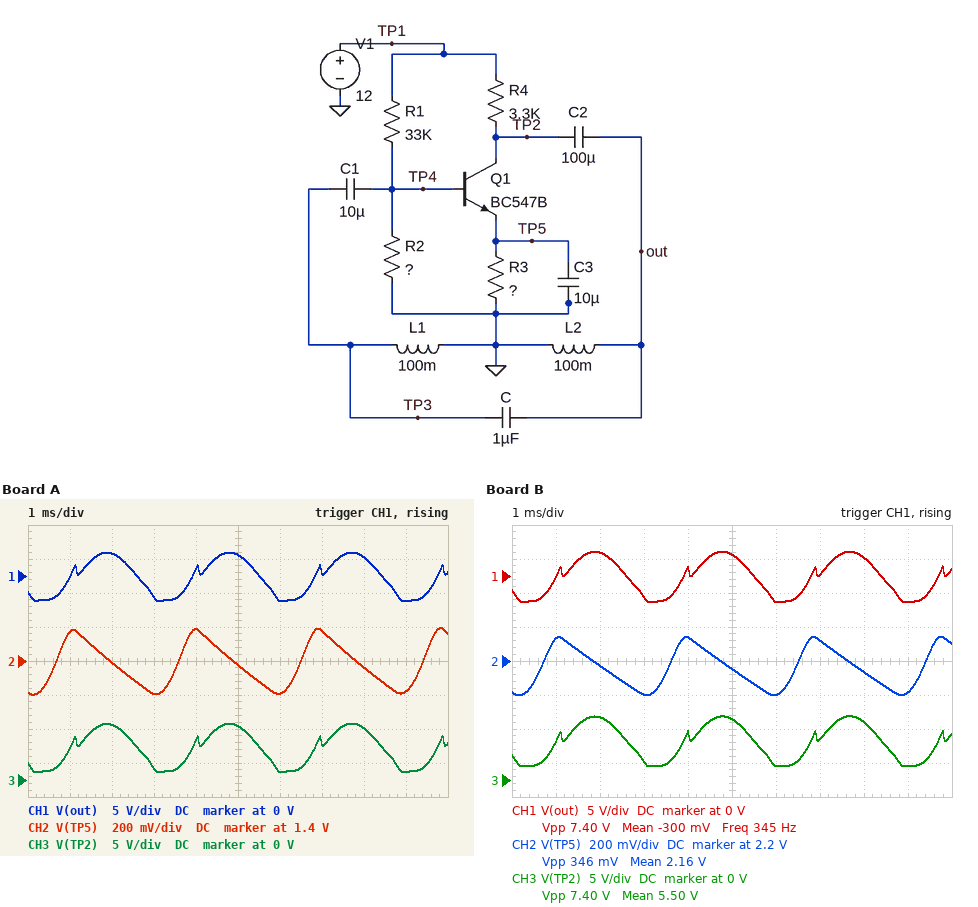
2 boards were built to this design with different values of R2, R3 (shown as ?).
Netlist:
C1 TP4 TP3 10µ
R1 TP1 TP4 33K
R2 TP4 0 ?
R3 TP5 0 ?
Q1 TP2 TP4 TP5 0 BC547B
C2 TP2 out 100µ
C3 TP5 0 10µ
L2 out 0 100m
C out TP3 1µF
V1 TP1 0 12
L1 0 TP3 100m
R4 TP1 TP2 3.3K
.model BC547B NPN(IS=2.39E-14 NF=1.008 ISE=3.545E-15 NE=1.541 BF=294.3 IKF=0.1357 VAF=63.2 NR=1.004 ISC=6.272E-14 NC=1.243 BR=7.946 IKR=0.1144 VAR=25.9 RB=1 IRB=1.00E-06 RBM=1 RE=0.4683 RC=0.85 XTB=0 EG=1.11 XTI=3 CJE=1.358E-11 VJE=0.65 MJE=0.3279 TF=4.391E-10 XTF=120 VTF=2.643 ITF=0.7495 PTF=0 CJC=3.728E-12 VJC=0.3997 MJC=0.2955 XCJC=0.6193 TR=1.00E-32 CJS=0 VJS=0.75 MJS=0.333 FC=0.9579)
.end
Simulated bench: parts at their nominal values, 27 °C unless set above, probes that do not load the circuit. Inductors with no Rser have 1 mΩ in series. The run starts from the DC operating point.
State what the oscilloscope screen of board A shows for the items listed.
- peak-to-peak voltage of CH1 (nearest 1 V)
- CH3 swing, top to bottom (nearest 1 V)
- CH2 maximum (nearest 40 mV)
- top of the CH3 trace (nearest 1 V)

7 V
7 V
1.60 V
8 V
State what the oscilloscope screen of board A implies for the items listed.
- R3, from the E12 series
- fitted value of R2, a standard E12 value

680 Ω
8.2 kΩ
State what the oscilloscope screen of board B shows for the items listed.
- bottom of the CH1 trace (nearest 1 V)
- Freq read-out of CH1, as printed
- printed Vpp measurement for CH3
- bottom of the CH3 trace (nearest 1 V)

-4 V
345 Hz
7.40 V
2 V
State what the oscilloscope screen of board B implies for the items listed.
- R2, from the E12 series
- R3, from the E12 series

12 kΩ
1.2 kΩ
